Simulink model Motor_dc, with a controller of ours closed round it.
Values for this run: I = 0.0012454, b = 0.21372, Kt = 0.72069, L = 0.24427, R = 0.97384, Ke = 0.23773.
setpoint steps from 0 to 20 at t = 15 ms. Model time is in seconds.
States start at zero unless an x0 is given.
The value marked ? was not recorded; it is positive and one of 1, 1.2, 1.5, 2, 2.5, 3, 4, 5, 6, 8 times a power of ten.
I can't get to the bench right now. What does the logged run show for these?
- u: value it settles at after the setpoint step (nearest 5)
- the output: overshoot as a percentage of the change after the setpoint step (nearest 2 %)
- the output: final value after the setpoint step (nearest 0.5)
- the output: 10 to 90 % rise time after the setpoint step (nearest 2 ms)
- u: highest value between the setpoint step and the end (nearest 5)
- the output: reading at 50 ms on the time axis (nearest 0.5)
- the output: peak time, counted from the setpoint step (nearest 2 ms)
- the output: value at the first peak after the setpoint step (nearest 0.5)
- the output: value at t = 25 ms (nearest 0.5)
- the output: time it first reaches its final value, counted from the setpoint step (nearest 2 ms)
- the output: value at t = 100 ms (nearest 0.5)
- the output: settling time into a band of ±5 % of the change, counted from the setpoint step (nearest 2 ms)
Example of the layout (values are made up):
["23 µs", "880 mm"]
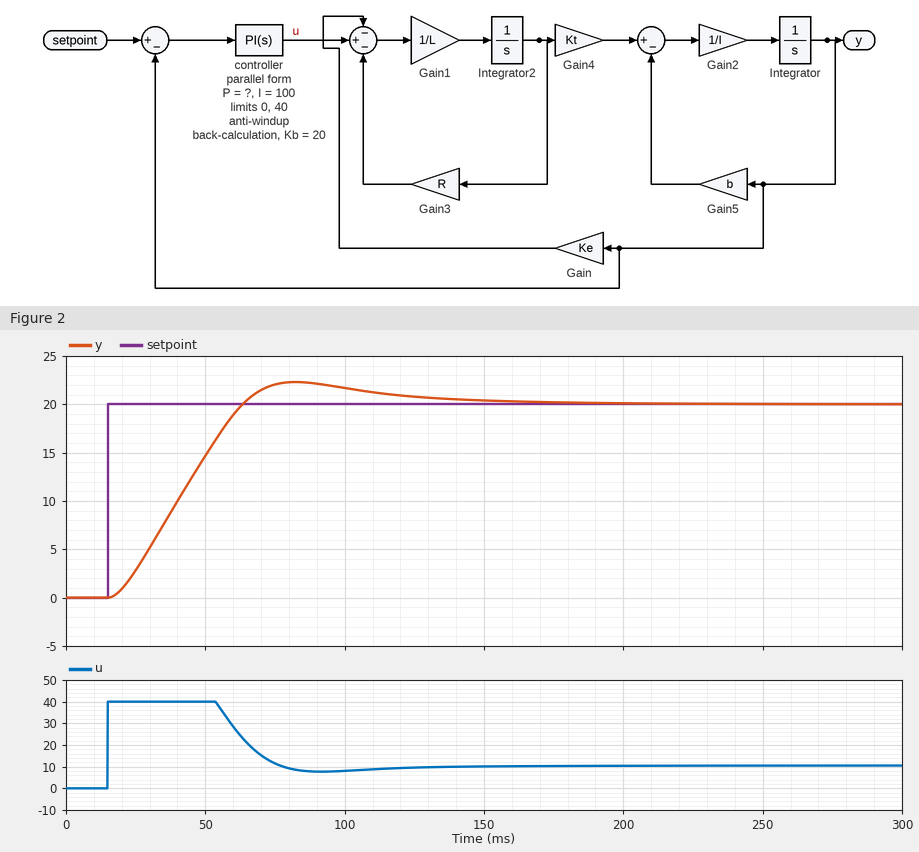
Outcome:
["10", "12 %", "20.0", "34 ms", "40", "14.5", "68 ms", "22.5", "3.0", "48 ms", "21.5", "102 ms"]
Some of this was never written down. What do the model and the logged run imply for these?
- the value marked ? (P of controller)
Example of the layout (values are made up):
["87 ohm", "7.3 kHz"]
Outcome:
["5"]
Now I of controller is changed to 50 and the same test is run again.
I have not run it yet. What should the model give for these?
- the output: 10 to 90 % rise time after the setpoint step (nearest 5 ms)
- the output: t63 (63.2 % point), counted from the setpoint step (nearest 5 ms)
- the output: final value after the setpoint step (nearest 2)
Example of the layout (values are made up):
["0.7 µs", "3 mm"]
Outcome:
["40 ms", "30 ms", "20"]
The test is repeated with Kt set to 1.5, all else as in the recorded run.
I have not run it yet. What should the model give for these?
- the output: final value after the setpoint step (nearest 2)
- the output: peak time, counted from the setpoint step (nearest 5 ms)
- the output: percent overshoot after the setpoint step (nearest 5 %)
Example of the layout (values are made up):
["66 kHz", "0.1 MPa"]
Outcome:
["20", "35 ms", "15 %"]
